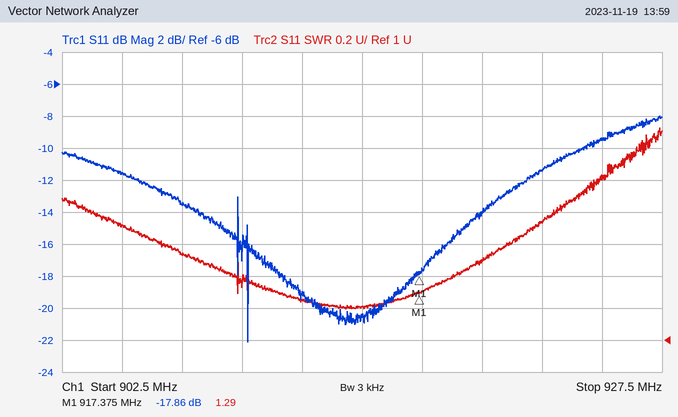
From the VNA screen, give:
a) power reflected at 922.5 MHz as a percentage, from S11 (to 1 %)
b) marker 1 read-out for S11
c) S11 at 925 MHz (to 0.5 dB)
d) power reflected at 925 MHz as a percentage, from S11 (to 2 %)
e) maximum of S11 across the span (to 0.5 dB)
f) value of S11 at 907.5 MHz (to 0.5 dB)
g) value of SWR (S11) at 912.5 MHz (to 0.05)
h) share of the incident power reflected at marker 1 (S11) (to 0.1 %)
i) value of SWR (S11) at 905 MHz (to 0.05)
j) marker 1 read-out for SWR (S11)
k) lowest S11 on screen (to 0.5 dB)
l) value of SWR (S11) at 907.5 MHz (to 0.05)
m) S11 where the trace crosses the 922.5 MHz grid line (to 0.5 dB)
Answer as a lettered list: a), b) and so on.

a) 7 %
b) -17.86 dB
c) -9.5 dB
d) 12 %
e) -8.0 dB
f) -13.5 dB
g) 1.25
h) 1.6 %
i) 1.70
j) 1.29
k) -22.0 dB
l) 1.55
m) -11.5 dB
